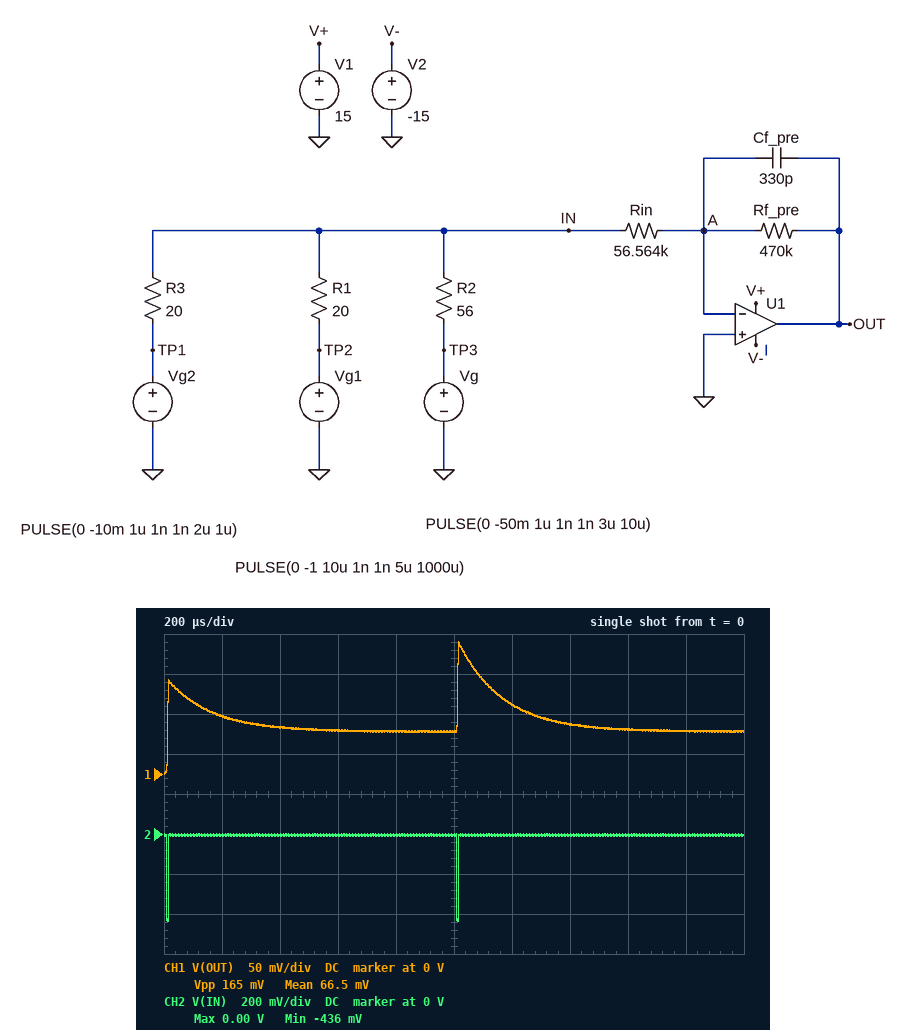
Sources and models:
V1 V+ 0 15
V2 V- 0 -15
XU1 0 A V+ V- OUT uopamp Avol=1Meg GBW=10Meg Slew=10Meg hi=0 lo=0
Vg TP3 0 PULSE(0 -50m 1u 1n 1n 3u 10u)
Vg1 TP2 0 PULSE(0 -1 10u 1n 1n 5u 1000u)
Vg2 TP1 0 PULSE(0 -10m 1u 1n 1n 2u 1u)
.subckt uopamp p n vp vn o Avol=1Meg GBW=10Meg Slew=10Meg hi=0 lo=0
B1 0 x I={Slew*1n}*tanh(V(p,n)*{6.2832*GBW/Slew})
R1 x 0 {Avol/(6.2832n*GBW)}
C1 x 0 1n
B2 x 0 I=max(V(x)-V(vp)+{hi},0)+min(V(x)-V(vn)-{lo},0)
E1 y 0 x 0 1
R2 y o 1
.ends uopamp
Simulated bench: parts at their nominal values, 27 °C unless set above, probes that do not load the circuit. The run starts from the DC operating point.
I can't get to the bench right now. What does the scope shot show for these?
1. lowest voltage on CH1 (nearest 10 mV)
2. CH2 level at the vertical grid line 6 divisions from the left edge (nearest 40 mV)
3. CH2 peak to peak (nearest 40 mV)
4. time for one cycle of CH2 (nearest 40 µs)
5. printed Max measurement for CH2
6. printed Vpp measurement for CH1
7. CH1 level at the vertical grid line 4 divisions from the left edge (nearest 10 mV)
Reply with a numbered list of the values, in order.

1. 0 V
2. 0 V
3. 440 mV
4. 1.00 ms
5. 0.00 V
6. 165 mV
7. 50 mV
